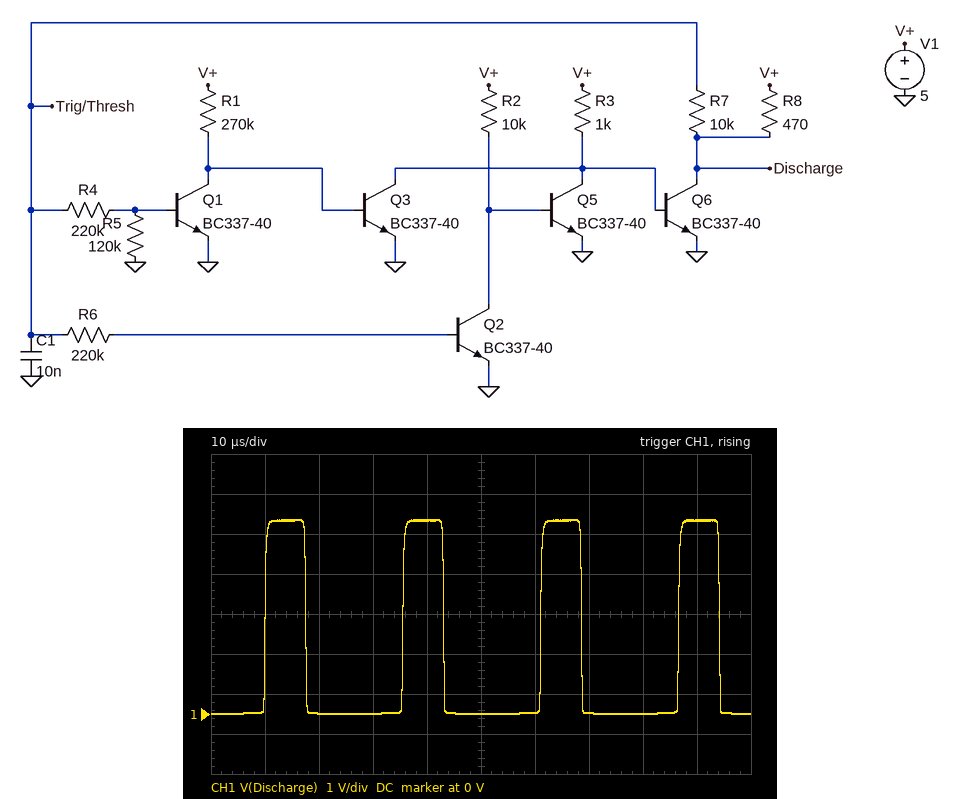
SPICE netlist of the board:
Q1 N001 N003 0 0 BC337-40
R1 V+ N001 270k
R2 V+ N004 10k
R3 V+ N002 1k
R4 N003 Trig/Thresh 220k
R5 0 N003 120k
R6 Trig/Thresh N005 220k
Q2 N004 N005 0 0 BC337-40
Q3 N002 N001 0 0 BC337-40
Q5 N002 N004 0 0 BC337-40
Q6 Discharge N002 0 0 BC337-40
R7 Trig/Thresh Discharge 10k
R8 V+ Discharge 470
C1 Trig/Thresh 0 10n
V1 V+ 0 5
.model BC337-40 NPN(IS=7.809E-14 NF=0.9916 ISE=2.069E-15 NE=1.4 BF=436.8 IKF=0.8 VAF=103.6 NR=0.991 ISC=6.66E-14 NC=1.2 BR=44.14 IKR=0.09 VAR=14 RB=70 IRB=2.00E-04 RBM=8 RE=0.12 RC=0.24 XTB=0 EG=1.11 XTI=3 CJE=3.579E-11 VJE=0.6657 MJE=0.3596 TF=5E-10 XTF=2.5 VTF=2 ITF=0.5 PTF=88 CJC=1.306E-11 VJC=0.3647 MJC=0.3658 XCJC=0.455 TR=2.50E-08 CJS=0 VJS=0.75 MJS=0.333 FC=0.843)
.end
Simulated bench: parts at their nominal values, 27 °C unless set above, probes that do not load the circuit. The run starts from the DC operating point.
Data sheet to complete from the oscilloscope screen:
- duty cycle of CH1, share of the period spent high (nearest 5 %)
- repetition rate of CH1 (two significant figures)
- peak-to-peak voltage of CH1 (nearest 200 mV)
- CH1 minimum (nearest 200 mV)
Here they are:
30 %
39 kHz
4.8 V
0 V
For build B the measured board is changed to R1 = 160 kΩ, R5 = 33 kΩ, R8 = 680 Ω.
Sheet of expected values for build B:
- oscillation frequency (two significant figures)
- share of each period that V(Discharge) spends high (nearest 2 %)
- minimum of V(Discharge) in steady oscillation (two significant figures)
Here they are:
43 kHz
82 %
15 mV
